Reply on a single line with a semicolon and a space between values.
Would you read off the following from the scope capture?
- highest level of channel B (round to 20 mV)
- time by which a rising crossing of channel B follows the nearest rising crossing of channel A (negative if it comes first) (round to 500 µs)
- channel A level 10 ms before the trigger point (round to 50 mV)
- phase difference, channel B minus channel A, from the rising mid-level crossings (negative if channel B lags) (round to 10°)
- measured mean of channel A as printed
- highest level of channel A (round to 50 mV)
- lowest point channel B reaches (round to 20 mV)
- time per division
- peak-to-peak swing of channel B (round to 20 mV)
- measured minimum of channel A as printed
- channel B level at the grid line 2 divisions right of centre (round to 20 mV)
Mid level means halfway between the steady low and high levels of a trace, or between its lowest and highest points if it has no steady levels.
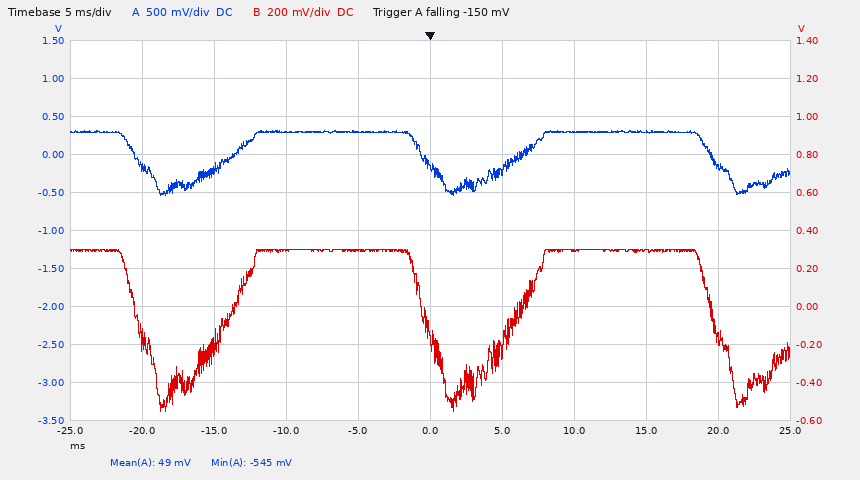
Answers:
300 mV; 0.0 ms; 300 mV; 0°; 49 mV; 300 mV; -560 mV; 5 ms; 860 mV; -545 mV; 300 mV
